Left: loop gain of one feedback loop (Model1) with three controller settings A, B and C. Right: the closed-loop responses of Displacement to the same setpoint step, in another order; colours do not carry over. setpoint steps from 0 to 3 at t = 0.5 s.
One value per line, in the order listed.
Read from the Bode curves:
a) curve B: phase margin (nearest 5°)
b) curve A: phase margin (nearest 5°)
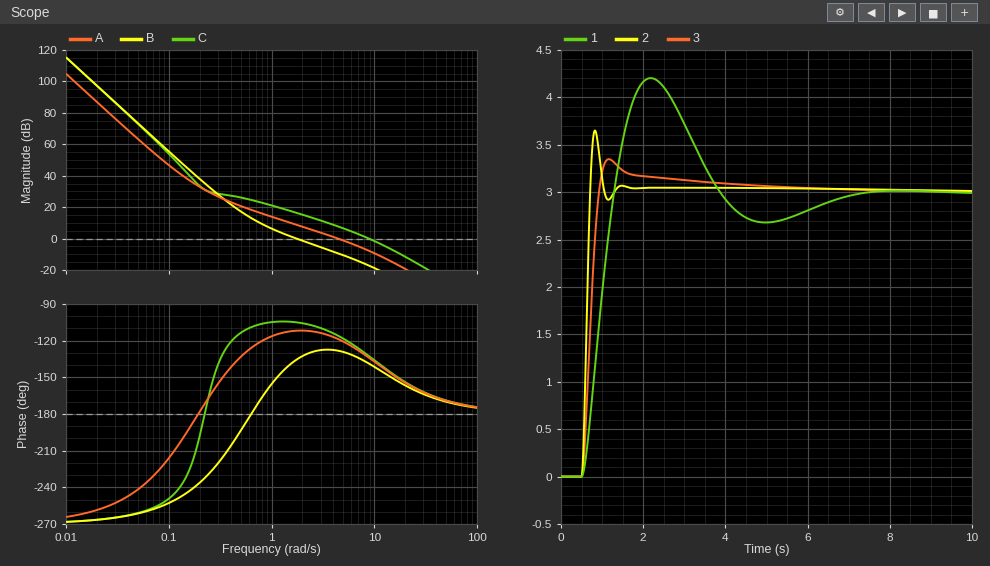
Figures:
45°
60°
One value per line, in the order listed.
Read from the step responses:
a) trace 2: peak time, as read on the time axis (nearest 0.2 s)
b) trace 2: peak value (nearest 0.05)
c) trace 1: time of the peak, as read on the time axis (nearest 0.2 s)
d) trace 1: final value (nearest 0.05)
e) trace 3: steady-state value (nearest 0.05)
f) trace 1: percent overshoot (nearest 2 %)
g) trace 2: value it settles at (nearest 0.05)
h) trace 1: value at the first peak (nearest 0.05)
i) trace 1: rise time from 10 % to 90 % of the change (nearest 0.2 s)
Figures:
0.8 s
3.65
2.2 s
3.00
3.00
40 %
3.00
4.20
0.6 s
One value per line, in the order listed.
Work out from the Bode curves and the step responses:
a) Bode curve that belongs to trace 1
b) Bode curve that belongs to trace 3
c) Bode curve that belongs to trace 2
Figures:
B
A
C
